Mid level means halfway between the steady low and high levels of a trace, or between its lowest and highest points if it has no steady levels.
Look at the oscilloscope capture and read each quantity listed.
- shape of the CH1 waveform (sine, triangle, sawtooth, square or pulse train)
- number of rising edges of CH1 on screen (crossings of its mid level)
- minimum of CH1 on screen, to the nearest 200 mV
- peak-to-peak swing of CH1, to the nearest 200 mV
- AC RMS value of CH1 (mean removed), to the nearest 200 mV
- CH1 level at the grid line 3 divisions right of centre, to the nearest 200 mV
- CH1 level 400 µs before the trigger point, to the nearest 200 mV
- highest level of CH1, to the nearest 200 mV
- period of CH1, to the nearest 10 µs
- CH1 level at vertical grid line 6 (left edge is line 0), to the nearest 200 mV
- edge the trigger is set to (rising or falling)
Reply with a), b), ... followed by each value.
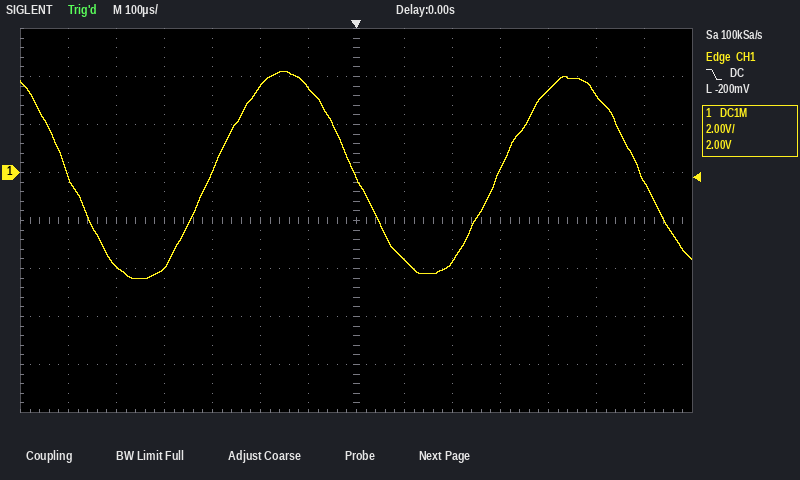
a) sine
b) 2
c) -4.4 V
d) 8.6 V
e) 3.0 V
f) 200 mV
g) -4.0 V
h) 4.2 V
i) 600 µs
j) 3.6 V
k) falling
